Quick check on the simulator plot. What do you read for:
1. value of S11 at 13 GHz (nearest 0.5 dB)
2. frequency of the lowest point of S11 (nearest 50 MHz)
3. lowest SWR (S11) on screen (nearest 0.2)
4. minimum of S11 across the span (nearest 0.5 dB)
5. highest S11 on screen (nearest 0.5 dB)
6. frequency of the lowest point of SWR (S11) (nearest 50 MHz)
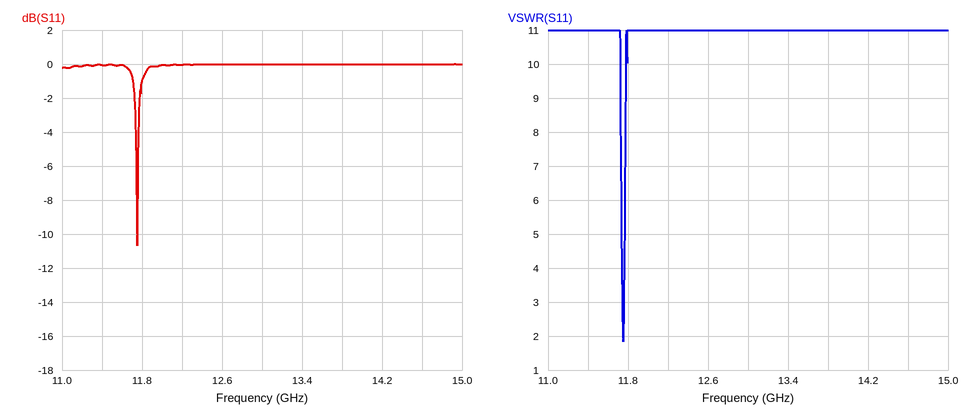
0.0 dB
11.75 GHz
1.8
-10.5 dB
0.0 dB
11.75 GHz
